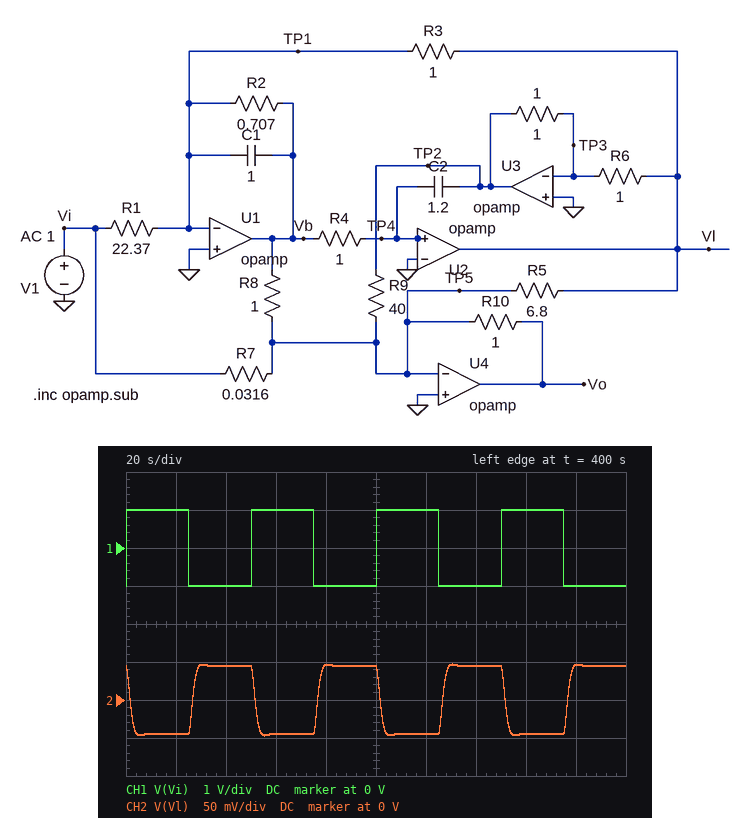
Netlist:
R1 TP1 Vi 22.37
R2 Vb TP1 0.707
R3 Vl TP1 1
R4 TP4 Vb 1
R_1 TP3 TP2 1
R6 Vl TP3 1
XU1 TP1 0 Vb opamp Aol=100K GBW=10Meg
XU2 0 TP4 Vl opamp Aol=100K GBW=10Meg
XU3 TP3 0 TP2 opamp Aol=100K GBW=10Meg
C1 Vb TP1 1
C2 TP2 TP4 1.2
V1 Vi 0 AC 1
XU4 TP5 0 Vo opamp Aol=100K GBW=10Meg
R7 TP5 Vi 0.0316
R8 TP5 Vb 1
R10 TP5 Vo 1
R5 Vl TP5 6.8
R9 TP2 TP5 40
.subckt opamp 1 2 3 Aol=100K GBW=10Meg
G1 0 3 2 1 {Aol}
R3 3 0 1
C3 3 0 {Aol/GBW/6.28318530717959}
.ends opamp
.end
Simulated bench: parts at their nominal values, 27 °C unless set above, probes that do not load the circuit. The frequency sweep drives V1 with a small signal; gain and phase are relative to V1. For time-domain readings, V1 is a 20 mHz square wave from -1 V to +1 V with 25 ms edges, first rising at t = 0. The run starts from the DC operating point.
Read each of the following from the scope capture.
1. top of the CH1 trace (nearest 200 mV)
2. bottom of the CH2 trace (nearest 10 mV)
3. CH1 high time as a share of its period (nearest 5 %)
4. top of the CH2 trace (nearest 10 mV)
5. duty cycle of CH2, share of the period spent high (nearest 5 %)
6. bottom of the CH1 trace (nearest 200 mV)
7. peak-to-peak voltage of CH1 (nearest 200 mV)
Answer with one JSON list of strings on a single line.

["1.0 V", "-50 mV", "50 %", "50 mV", "50 %", "-1.0 V", "2.0 V"]
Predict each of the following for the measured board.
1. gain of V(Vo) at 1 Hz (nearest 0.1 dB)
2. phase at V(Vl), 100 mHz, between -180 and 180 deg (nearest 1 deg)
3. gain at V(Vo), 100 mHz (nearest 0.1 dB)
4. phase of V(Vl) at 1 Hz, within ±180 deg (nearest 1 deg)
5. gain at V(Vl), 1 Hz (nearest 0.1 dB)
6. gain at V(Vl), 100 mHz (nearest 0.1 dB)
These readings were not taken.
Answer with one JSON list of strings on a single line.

["30.0 dB", "116 deg", "30.0 dB", "13 deg", "-60.5 dB", "-28.5 dB"]
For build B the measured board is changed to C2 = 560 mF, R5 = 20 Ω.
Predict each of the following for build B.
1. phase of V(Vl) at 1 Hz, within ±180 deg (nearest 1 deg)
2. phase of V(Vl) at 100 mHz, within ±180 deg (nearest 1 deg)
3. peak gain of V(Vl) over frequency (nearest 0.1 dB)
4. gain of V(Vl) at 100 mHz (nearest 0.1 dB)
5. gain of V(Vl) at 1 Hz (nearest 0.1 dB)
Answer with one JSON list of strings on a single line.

["13 deg", "147 deg", "-26.1 dB", "-26.3 dB", "-53.7 dB"]
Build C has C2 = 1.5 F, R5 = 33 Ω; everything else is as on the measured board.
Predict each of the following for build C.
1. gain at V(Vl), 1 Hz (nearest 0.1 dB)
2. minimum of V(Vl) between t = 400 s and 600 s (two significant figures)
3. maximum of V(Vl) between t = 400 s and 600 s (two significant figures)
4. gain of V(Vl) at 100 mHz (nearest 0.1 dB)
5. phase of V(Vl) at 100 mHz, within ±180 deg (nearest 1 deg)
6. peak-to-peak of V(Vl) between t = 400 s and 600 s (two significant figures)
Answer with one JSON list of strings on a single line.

["-62.5 dB", "-45 mV", "45 mV", "-29.9 dB", "107 deg", "90 mV"]
